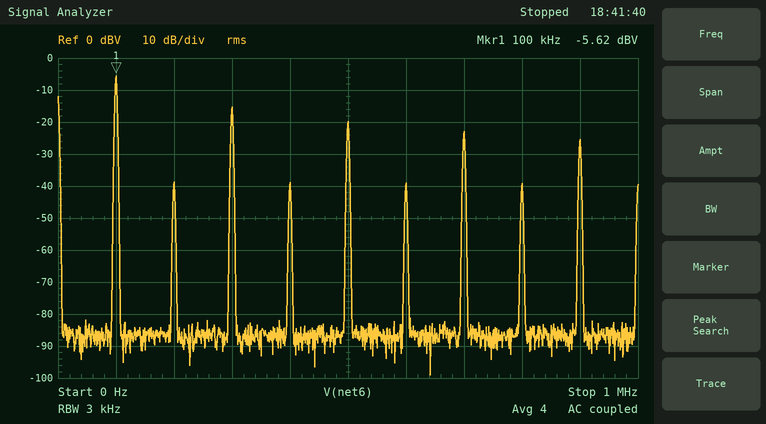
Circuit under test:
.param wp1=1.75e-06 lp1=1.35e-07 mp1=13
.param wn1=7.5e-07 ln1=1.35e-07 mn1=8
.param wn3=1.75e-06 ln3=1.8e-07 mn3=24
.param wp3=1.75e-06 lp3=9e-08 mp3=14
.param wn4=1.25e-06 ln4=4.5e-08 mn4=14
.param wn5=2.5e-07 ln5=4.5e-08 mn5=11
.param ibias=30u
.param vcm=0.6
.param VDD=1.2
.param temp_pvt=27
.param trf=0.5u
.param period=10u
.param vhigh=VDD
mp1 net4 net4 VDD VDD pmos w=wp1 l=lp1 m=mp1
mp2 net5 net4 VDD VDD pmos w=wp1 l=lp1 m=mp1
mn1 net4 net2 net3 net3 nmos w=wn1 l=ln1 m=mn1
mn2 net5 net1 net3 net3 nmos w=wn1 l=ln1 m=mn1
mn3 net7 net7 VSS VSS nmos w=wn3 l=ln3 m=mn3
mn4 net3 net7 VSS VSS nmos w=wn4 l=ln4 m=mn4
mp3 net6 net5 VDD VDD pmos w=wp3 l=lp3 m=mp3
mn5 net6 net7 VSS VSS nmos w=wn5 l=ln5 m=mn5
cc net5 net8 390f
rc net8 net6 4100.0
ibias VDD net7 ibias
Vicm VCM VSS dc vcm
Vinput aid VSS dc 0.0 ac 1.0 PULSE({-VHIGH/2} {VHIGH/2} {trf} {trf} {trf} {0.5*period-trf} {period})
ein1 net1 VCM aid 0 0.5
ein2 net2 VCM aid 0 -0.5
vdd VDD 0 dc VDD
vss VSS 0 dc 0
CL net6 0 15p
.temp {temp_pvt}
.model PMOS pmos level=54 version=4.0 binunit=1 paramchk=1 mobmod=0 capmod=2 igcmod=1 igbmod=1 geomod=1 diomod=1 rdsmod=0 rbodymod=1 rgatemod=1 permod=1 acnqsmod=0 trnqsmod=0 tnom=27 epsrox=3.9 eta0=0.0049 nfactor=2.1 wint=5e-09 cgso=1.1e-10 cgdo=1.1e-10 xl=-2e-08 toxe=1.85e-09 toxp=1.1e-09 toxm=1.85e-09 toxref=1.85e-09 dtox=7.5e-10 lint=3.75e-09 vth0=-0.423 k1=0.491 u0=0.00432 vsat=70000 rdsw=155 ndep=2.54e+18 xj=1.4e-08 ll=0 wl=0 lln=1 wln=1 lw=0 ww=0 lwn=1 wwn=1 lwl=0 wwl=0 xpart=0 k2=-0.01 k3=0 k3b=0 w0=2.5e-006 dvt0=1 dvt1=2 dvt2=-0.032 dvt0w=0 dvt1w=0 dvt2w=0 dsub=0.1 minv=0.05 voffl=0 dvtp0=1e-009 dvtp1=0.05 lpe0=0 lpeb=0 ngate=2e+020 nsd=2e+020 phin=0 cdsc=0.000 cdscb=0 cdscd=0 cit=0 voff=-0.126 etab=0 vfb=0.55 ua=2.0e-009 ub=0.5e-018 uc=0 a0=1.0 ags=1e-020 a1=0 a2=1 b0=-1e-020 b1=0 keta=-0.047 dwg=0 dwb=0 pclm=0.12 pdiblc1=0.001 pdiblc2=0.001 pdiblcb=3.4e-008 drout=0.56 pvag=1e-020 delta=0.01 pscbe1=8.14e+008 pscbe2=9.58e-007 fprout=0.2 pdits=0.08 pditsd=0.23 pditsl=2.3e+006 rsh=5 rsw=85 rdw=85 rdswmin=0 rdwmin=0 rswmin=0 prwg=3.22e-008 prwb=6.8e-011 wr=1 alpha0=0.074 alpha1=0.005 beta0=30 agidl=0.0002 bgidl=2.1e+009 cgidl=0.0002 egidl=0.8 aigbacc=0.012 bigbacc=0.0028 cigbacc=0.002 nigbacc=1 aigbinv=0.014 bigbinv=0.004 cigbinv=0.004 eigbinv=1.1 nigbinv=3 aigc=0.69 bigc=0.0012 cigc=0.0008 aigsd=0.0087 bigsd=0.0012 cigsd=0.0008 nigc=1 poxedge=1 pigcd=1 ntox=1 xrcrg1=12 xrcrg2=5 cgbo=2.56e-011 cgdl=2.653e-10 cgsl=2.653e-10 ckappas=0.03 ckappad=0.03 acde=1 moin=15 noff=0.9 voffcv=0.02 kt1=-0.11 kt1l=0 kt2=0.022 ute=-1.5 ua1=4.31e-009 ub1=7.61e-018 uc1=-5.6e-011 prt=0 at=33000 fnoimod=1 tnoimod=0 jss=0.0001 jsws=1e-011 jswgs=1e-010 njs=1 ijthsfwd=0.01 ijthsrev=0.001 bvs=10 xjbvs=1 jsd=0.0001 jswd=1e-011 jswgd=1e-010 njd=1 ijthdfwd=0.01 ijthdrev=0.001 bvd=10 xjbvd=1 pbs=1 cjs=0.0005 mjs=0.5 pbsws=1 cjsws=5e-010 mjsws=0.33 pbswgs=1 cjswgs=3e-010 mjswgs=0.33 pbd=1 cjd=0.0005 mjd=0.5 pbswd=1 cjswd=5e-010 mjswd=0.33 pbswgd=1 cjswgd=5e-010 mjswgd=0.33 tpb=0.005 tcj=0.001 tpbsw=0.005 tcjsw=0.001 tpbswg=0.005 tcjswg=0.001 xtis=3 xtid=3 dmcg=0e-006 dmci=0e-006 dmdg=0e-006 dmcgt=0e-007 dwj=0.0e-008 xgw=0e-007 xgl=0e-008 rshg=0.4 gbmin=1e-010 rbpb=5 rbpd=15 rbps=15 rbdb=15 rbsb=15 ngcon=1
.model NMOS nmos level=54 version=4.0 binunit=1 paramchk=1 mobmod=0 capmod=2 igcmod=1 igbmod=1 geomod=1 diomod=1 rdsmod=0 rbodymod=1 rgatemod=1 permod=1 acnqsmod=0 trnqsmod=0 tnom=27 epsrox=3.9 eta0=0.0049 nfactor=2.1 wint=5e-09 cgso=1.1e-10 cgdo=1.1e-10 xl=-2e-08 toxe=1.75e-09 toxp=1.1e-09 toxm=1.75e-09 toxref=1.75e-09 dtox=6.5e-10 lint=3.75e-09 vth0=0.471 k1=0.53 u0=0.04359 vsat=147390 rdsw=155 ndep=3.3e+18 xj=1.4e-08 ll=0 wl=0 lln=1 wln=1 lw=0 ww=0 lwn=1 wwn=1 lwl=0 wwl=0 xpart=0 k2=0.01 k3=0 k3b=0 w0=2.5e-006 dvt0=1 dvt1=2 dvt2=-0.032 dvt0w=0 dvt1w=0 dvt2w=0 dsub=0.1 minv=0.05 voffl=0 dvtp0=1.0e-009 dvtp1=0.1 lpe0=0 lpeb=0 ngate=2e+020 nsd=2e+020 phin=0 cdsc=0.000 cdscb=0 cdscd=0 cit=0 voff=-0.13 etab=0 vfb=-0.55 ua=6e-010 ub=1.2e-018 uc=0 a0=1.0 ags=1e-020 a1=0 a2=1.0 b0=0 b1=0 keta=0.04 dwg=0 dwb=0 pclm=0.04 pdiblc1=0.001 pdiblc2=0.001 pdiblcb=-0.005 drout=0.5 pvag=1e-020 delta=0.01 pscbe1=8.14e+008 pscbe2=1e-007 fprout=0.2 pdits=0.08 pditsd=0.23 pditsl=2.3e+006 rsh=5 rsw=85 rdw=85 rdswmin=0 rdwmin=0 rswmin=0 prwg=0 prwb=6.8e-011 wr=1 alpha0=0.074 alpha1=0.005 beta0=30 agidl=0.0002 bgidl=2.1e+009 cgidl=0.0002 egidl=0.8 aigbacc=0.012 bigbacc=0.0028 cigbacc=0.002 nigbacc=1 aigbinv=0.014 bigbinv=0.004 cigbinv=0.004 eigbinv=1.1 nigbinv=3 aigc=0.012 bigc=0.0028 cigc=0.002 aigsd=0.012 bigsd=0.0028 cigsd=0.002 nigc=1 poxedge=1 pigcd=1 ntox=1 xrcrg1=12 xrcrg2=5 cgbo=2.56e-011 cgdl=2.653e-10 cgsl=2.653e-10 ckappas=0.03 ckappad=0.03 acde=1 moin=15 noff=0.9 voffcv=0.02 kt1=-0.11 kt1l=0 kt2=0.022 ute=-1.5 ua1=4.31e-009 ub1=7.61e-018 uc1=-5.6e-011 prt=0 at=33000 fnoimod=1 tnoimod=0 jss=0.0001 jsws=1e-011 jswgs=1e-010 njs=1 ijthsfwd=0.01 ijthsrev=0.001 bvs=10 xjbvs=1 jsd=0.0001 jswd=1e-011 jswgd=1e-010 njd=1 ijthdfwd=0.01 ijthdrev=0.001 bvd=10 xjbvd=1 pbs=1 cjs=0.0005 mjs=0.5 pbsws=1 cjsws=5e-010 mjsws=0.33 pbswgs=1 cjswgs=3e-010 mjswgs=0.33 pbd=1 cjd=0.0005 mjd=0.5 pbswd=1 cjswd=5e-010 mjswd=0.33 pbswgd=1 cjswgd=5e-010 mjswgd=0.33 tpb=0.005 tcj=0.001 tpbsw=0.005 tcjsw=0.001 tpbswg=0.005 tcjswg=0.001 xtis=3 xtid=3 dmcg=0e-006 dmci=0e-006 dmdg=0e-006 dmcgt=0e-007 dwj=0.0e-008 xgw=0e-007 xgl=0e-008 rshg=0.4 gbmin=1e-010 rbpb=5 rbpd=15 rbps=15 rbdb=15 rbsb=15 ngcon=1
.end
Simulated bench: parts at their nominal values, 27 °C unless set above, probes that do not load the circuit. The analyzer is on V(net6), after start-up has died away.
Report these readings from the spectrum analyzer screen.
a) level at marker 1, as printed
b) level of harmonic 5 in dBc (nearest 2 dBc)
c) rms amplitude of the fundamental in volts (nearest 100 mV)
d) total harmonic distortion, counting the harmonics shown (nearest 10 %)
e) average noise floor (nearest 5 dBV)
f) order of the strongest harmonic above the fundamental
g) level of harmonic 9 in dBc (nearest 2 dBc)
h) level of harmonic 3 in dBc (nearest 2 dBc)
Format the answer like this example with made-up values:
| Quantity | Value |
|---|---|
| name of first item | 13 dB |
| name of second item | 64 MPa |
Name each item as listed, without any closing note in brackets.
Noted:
| Quantity | Value |
|---|---|
| level at marker 1, as printed | -5.62 dBV |
| level of harmonic 5 in dBc | -14 dBc |
| rms amplitude of the fundamental in volts | 500 mV |
| total harmonic distortion, counting the harmonics shown | 40 % |
| average noise floor | -85 dBV |
| order of the strongest harmonic above the fundamental | 3 |
| level of harmonic 9 in dBc | -20 dBc |
| level of harmonic 3 in dBc | -10 dBc |
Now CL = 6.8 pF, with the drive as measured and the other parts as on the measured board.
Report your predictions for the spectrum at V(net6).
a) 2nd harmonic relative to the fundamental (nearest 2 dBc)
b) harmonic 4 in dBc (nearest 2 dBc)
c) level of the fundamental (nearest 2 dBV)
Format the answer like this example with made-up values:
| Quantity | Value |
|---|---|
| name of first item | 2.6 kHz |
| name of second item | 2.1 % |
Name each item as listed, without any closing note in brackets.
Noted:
| Quantity | Value |
|---|---|
| 2nd harmonic relative to the fundamental | -40 dBc |
| harmonic 4 in dBc | -40 dBc |
| level of the fundamental | -6 dBV |
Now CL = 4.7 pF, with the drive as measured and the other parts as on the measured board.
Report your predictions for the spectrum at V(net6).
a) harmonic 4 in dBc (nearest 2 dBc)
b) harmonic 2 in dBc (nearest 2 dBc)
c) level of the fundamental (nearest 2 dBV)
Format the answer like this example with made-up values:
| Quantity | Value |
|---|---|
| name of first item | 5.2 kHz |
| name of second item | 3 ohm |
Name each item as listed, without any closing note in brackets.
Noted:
| Quantity | Value |
|---|---|
| harmonic 4 in dBc | -44 dBc |
| harmonic 2 in dBc | -44 dBc |
| level of the fundamental | -6 dBV |
